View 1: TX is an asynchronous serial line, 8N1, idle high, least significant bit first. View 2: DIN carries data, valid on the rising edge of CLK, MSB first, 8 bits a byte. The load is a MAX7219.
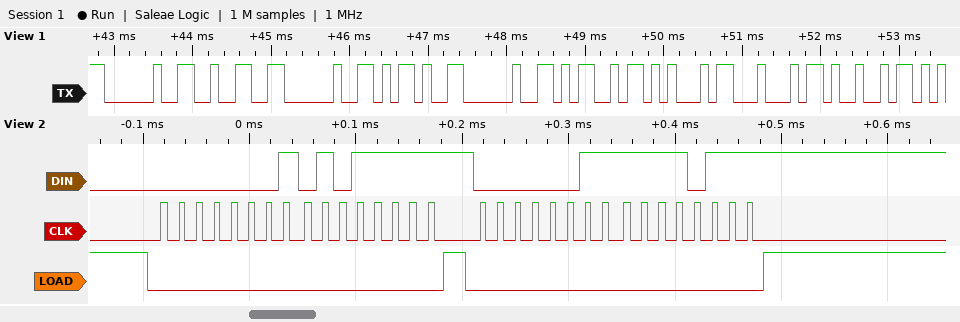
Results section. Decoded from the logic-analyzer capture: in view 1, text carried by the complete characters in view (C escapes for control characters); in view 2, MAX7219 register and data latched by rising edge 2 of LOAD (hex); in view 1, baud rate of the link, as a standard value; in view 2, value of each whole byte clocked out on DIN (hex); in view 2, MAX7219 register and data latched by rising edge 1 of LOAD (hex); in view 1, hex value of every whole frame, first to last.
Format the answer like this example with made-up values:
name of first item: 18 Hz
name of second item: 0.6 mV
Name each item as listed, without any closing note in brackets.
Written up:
in view 1, text carried by the complete characters in view: " 2 - MEDI"
in view 2, MAX7219 register and data latched by rising edge 2 of LOAD: register 0x3, data 0xF7
in view 1, baud rate of the link, as a standard value: 9600 baud
in view 2, value of each whole byte clocked out on DIN: 01 5F 03 F7
in view 2, MAX7219 register and data latched by rising edge 1 of LOAD: register 0x1, data 0x5F
in view 1, hex value of every whole frame, first to last: 0x20 0x32 0x20 0x2D 0x20 0x4D 0x45 0x44 0x49
